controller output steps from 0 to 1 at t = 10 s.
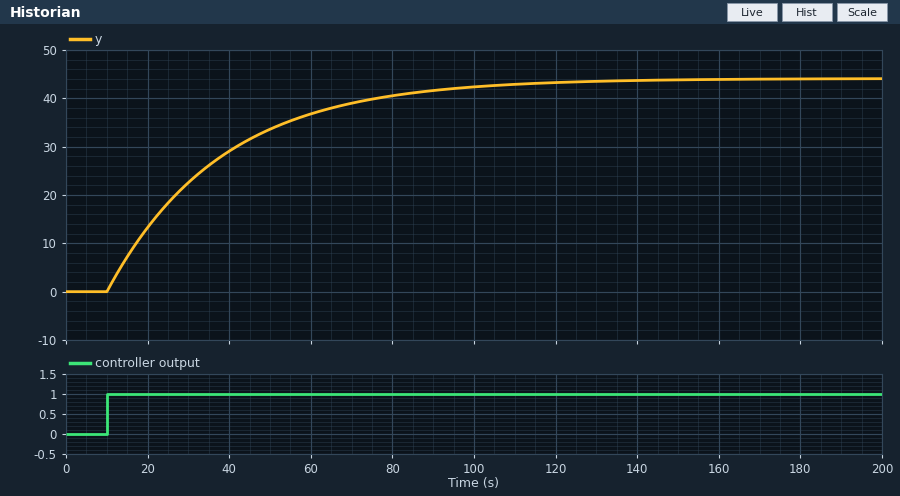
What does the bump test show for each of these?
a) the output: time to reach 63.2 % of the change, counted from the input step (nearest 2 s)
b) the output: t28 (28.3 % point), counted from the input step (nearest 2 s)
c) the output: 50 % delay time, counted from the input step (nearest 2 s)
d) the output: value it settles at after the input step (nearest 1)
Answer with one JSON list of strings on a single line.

["28 s", "10 s", "20 s", "44"]
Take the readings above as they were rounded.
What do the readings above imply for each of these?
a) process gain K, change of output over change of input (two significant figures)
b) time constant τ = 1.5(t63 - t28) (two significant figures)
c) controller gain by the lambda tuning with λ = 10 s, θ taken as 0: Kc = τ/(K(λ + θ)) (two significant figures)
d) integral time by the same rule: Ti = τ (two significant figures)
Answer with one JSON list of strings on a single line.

["44", "27 s", "0.061", "27 s"]
